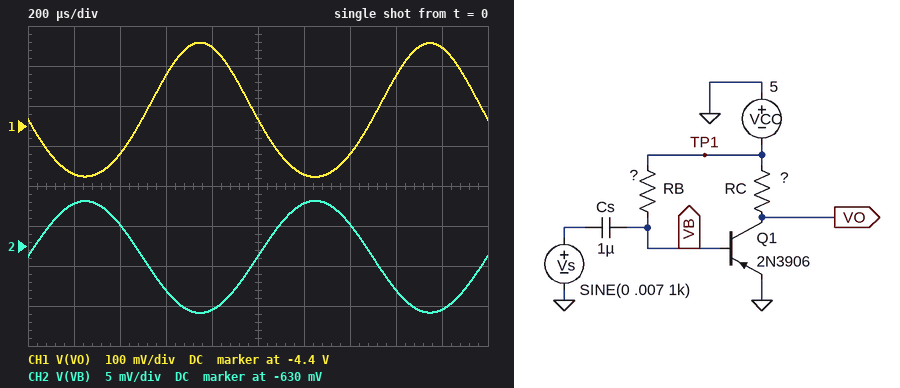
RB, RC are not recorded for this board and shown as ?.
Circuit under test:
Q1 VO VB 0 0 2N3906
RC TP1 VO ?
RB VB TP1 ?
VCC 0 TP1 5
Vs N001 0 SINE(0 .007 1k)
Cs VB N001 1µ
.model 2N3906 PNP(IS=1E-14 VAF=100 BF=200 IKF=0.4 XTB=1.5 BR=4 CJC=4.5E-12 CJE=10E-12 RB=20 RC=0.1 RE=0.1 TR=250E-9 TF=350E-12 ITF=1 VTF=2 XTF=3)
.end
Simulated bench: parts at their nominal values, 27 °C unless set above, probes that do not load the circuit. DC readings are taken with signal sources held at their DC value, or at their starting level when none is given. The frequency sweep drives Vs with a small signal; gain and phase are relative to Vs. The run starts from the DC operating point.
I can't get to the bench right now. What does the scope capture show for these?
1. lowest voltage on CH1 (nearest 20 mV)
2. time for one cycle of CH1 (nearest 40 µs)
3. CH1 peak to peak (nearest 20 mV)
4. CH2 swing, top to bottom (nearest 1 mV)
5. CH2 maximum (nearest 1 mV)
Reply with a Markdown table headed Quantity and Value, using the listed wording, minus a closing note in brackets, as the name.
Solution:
| Quantity | Value |
|---|---|
| lowest voltage on CH1 | -4.52 V |
| time for one cycle of CH1 | 1.00 ms |
| CH1 peak to peak | 340 mV |
| CH2 swing, top to bottom | 14 mV |
| CH2 maximum | -624 mV |
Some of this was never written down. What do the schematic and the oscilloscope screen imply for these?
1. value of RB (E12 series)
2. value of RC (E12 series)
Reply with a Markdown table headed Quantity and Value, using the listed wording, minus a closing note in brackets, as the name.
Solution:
| Quantity | Value |
|---|---|
| value of RB | 2.2 MΩ |
| value of RC | 1.5 kΩ |
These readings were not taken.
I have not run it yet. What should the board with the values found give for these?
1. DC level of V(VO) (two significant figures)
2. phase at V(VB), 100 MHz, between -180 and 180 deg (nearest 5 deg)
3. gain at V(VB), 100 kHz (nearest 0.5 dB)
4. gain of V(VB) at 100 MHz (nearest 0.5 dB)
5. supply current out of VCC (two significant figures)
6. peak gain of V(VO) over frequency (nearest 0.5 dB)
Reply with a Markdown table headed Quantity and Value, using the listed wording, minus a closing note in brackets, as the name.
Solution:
| Quantity | Value |
|---|---|
| DC level of V(VO) | -4.4 V |
| phase at V(VB), 100 MHz, between -180 and 180 deg | 0 deg |
| gain at V(VB), 100 kHz | 0 dB |
| gain of V(VB) at 100 MHz | 0 dB |
| supply current out of VCC | 410 µA |
| peak gain of V(VO) over frequency | 27.5 dB |
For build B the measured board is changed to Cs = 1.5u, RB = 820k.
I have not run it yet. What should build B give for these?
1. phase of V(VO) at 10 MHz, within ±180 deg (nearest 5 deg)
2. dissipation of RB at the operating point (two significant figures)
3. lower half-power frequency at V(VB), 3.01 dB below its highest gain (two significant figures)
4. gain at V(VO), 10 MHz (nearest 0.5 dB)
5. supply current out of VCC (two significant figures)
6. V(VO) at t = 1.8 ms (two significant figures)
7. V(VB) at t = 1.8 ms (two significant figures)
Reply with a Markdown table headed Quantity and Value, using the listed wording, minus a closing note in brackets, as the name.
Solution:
| Quantity | Value |
|---|---|
| phase of V(VO) at 10 MHz, within ±180 deg | 155 deg |
| dissipation of RB at the operating point | 23 µW |
| lower half-power frequency at V(VB), 3.01 dB below its highest gain | 22 Hz |
| gain at V(VO), 10 MHz | 35.0 dB |
| supply current out of VCC | 1.1 mA |
| V(VO) at t = 1.8 ms | -2.9 V |
| V(VB) at t = 1.8 ms | -660 mV |
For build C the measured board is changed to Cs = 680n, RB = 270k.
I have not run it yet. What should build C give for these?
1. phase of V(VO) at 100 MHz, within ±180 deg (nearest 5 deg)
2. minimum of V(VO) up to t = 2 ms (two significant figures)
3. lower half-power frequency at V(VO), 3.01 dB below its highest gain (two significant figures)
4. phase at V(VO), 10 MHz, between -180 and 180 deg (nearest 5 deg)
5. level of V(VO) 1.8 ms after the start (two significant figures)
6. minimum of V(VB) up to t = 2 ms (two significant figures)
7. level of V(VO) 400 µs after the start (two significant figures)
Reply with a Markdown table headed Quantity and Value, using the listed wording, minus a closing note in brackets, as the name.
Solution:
| Quantity | Value |
|---|---|
| phase of V(VO) at 100 MHz, within ±180 deg | 80 deg |
| minimum of V(VO) up to t = 2 ms | -1.8 V |
| lower half-power frequency at V(VO), 3.01 dB below its highest gain | 180 Hz |
| phase at V(VO), 10 MHz, between -180 and 180 deg | 115 deg |
| level of V(VO) 1.8 ms after the start | -170 mV |
| minimum of V(VB) up to t = 2 ms | -690 mV |
| level of V(VO) 400 µs after the start | -700 mV |
